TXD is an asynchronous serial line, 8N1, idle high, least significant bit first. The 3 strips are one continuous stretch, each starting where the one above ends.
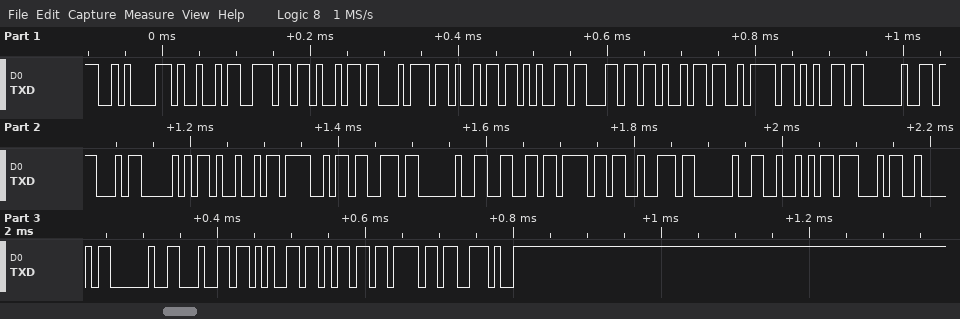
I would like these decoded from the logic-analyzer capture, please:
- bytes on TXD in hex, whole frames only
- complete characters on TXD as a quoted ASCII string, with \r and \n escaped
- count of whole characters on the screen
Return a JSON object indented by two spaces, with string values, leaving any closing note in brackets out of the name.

{
  "bytes on TXD in hex, whole frames only": "0A 49 6E 69 74 69 65 6C 69 7A 65 20 47 50 49 4F 73 20 66 6F 72 20 52 47 42 20 64 65 6D 6F 2E",
  "complete characters on TXD as a quoted ASCII string, with \\r and \\n escaped": "\"\\nInitielize GPIOs for RGB demo.\"",
  "count of whole characters on the screen": "31"
}
